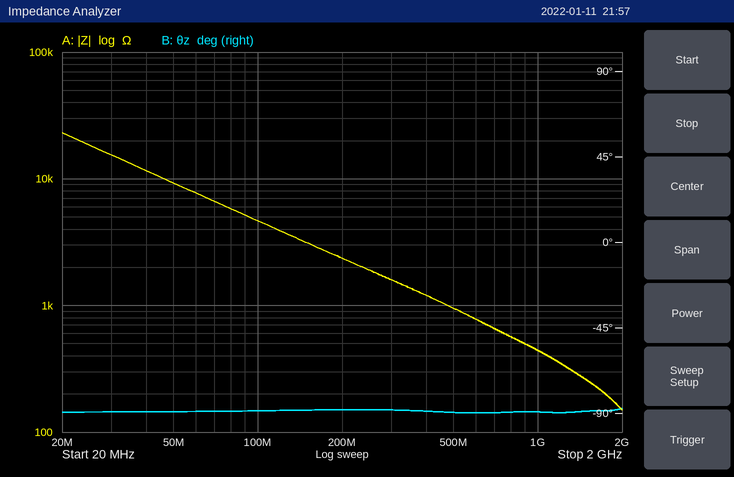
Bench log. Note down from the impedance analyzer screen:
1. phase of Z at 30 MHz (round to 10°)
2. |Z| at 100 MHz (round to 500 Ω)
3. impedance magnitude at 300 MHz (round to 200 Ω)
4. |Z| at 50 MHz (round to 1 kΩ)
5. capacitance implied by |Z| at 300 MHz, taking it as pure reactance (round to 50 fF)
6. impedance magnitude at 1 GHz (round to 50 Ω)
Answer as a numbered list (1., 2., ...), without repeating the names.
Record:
1. -90°
2. 4.5 kΩ
3. 1.6 kΩ
4. 9 kΩ
5. 350 fF
6. 450 Ω
